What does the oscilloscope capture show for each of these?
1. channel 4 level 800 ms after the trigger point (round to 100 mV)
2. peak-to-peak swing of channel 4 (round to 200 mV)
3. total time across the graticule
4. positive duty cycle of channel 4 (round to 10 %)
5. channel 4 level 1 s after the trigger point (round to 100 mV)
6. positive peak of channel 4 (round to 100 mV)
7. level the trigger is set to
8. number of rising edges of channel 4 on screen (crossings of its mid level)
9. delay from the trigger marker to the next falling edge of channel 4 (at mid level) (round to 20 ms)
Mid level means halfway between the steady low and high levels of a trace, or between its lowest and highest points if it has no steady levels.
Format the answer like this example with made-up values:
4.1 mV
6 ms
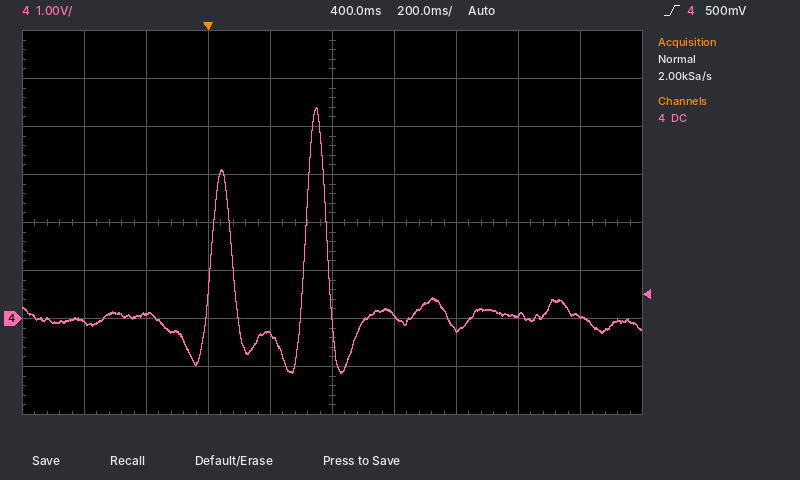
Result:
-200 mV
5.6 V
2 s
20 %
100 mV
4.4 V
500 mV
2
80 ms
